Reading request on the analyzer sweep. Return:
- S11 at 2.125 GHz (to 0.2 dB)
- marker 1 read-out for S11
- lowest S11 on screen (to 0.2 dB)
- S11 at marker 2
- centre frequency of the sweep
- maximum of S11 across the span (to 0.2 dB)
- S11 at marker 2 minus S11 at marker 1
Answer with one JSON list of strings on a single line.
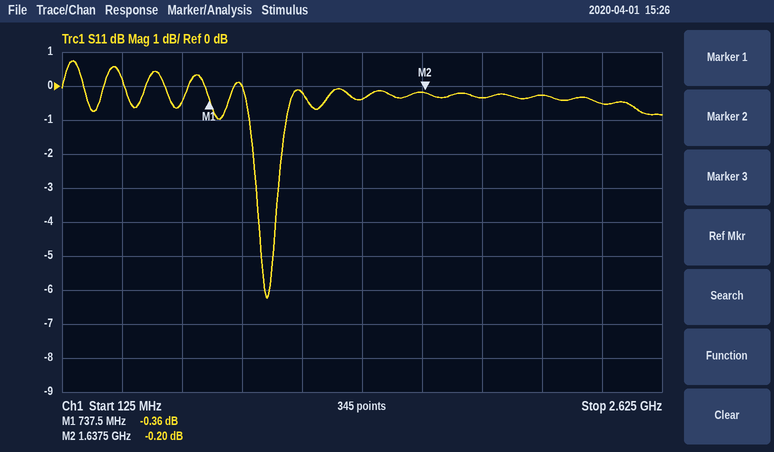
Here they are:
["-0.2 dB", "-0.36 dB", "-6.2 dB", "-0.20 dB", "1.375 GHz", "0.8 dB", "0.16 dB"]
